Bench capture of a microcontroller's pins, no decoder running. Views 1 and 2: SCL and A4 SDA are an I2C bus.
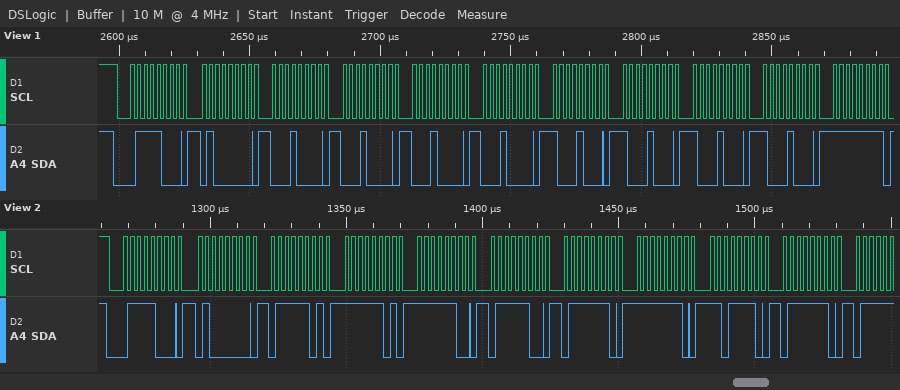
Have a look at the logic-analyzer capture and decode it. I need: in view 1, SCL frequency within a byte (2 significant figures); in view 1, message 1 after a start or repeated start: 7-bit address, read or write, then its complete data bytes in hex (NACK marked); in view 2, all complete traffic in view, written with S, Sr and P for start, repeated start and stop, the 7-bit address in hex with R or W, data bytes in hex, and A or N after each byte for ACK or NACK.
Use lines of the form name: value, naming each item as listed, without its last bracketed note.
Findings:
in view 1, SCL frequency within a byte: 400 kHz
in view 1, message 1 after a start or repeated start: 7-bit address, read or write, then its complete data bytes in hex: 0x3C write: 40 10 10 10 10 88 88 88 88 FF
in view 2, all complete traffic in view, written with S, Sr and P for start, repeated start and stop, the 7-bit address in hex with R or W, data bytes in hex, and A or N after each byte for ACK or NACK: S 3CW A 40 A 7D A FD A FC A 7C A 7E A FE A DE A 7E A
